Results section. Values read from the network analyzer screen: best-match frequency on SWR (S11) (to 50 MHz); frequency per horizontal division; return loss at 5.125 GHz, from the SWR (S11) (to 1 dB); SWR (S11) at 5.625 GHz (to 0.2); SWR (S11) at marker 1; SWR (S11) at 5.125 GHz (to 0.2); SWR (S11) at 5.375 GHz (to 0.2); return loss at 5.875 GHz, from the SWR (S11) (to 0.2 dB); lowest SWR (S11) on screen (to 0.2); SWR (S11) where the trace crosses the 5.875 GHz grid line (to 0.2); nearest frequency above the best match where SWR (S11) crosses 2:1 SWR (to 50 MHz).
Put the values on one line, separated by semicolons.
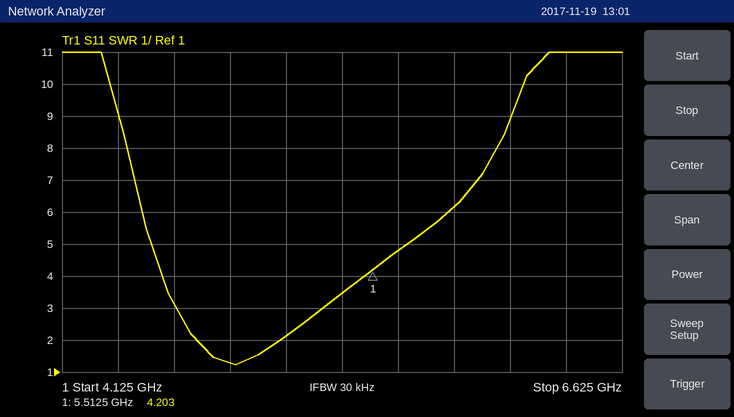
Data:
4.90 GHz; 250 MHz; 9 dB; 4.8; 4.203; 2.2; 3.4; 2.8 dB; 1.2; 6.2; 5.10 GHz
